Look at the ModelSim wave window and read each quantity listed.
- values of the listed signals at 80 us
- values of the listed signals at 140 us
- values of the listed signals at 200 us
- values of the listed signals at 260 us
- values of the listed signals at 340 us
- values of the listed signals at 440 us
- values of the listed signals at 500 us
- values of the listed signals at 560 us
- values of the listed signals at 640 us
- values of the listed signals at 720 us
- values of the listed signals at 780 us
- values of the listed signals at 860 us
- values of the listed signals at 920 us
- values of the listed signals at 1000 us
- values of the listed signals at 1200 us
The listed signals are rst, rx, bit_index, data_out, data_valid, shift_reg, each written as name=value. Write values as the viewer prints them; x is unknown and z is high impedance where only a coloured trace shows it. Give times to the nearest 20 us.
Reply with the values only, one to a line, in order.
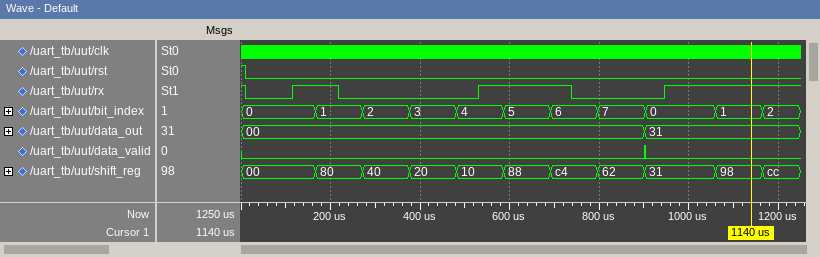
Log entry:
rst=0, rx=0, bit_index=0, data_out=00, data_valid=0, shift_reg=00
rst=0, rx=1, bit_index=0, data_out=00, data_valid=0, shift_reg=00
rst=0, rx=1, bit_index=1, data_out=00, data_valid=0, shift_reg=80
rst=0, rx=0, bit_index=1, data_out=00, data_valid=0, shift_reg=80
rst=0, rx=0, bit_index=2, data_out=00, data_valid=0, shift_reg=40
rst=0, rx=0, bit_index=3, data_out=00, data_valid=0, shift_reg=20
rst=0, rx=0, bit_index=4, data_out=00, data_valid=0, shift_reg=10
rst=0, rx=1, bit_index=4, data_out=00, data_valid=0, shift_reg=10
rst=0, rx=1, bit_index=5, data_out=00, data_valid=0, shift_reg=88
rst=0, rx=1, bit_index=6, data_out=00, data_valid=0, shift_reg=c4
rst=0, rx=0, bit_index=6, data_out=00, data_valid=0, shift_reg=c4
rst=0, rx=0, bit_index=7, data_out=00, data_valid=0, shift_reg=62
rst=0, rx=0, bit_index=0, data_out=31, data_valid=0, shift_reg=31
rst=0, rx=1, bit_index=0, data_out=31, data_valid=0, shift_reg=31
rst=0, rx=1, bit_index=2, data_out=31, data_valid=0, shift_reg=cc
